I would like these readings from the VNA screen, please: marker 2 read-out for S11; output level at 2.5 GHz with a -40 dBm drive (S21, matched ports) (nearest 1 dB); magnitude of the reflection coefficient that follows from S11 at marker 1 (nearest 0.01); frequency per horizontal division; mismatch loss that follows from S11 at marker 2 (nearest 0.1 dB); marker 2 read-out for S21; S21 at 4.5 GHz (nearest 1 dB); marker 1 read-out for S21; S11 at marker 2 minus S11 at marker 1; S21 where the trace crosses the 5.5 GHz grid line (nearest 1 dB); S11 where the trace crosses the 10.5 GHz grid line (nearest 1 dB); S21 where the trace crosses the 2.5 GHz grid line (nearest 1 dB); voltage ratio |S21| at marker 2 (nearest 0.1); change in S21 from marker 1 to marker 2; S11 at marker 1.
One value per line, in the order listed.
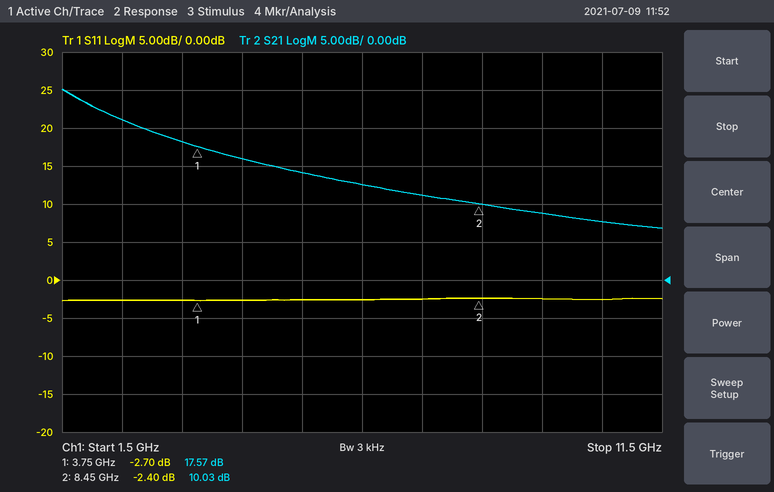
-2.40 dB
-19 dBm
0.73
1 GHz
3.7 dB
10.03 dB
16 dB
17.57 dB
0.30 dB
14 dB
-3 dB
21 dB
3.2
-7.54 dB
-2.70 dB
